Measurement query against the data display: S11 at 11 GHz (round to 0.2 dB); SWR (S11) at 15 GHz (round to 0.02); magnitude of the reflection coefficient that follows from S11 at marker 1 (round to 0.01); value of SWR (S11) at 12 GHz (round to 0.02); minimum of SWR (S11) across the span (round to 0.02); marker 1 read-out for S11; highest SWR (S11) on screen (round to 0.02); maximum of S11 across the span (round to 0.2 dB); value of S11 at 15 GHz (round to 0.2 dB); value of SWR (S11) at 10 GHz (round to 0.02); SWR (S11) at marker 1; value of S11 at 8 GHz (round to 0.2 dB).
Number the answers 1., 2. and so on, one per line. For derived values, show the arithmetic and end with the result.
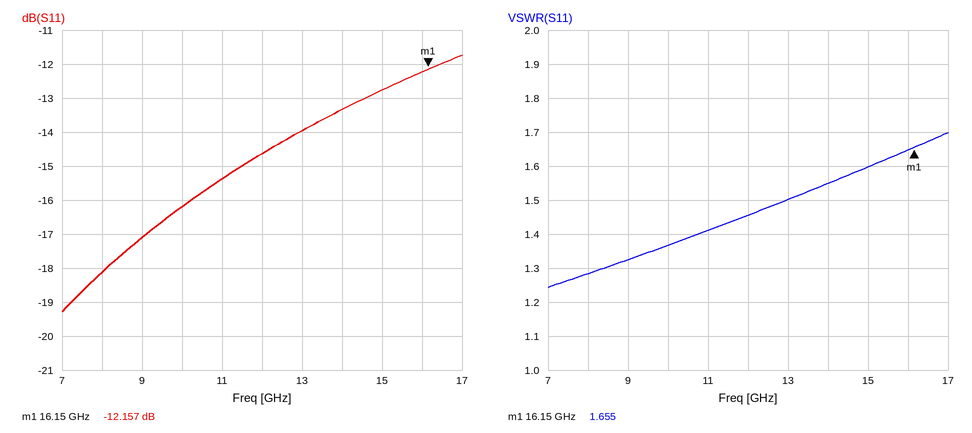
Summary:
1. -15.4 dB
2. 1.60
3. 10^(-12.157/20) ≈ 0.25
4. 1.46
5. 1.24
6. -12.157 dB
7. 1.70
8. -11.8 dB
9. -12.8 dB
10. 1.36
11. 1.655
12. -18.2 dB
